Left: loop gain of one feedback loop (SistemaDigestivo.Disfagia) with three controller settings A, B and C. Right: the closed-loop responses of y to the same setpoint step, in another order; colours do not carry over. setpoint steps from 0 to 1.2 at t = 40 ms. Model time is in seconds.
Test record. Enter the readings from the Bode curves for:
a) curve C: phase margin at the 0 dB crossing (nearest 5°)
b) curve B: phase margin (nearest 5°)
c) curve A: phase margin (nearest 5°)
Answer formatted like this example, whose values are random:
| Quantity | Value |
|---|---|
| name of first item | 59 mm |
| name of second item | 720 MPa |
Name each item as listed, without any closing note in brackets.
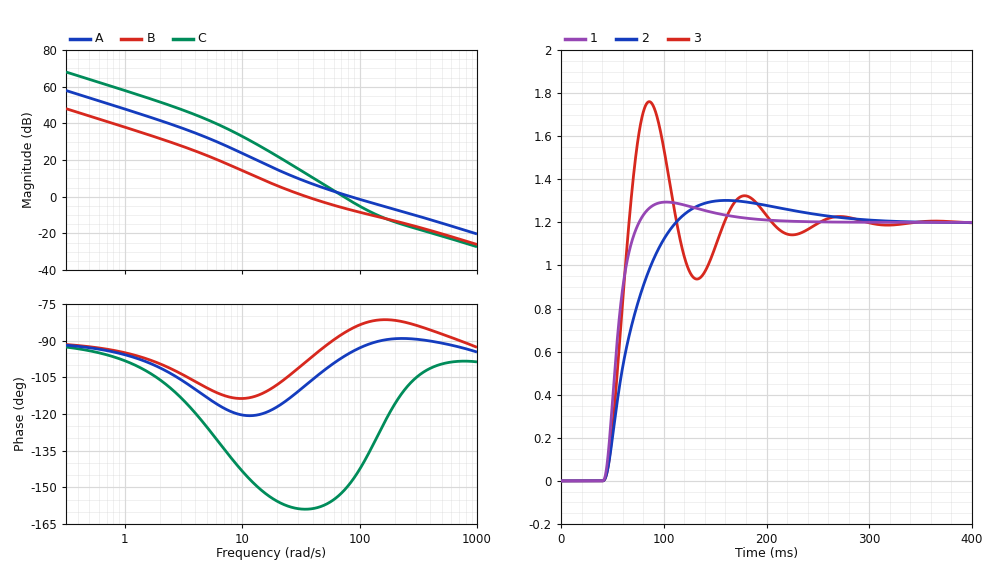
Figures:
| Quantity | Value |
|---|---|
| curve C: phase margin at the 0 dB crossing | 30° |
| curve B: phase margin | 80° |
| curve A: phase margin | 85° |
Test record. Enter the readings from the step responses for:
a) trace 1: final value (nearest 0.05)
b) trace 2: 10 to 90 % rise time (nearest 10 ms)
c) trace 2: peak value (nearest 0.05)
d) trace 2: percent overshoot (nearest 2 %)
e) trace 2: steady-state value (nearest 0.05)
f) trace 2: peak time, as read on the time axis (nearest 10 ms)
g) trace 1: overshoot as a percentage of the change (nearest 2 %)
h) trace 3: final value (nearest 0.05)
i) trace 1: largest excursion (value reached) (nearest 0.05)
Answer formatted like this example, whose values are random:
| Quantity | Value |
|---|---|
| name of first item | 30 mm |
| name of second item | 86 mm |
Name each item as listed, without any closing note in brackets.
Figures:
| Quantity | Value |
|---|---|
| trace 1: final value | 1.20 |
| trace 2: 10 to 90 % rise time | 50 ms |
| trace 2: peak value | 1.30 |
| trace 2: percent overshoot | 8 % |
| trace 2: steady-state value | 1.20 |
| trace 2: peak time, as read on the time axis | 160 ms |
| trace 1: overshoot as a percentage of the change | 8 % |
| trace 3: final value | 1.20 |
| trace 1: largest excursion (value reached) | 1.30 |
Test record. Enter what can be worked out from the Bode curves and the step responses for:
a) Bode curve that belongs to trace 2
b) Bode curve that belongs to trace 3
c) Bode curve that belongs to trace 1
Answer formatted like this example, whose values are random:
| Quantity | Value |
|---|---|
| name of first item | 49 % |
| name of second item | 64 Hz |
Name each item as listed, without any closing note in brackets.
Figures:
| Quantity | Value |
|---|---|
| Bode curve that belongs to trace 2 | B |
| Bode curve that belongs to trace 3 | C |
| Bode curve that belongs to trace 1 | A |
